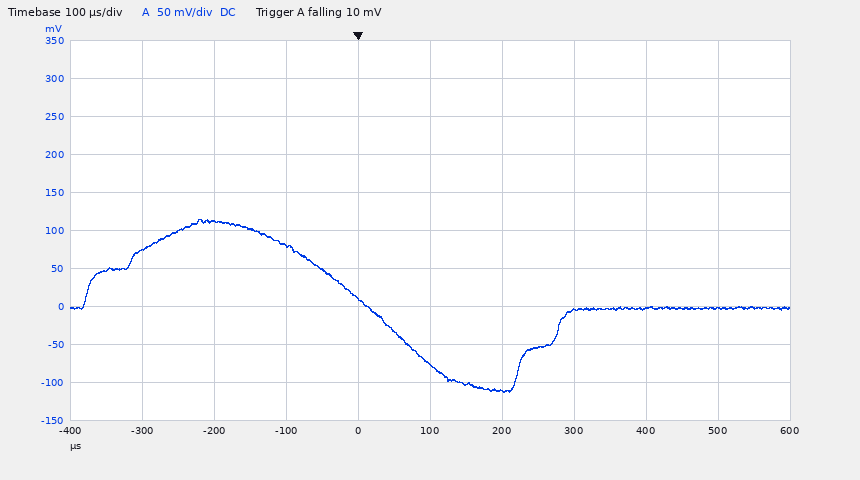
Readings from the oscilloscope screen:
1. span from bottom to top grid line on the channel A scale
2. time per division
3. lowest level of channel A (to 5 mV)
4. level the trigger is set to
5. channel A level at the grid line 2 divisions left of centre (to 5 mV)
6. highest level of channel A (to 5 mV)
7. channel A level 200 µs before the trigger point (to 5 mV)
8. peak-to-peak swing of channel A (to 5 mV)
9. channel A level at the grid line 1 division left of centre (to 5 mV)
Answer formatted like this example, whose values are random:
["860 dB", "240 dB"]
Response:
["500 mV", "100 µs", "-115 mV", "10 mV", "80 mV", "115 mV", "110 mV", "230 mV", "10 mV"]
